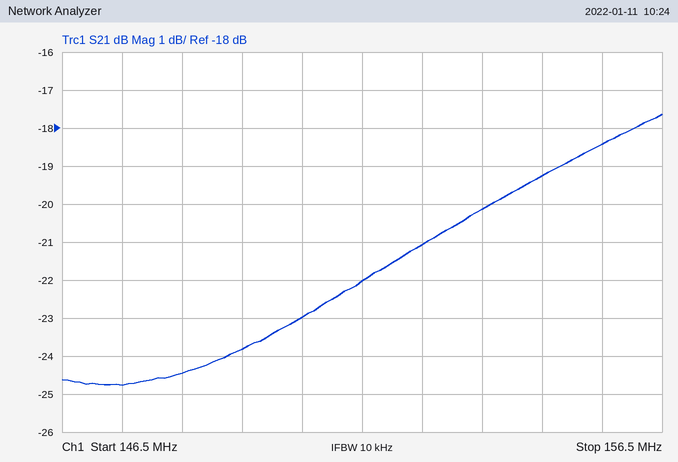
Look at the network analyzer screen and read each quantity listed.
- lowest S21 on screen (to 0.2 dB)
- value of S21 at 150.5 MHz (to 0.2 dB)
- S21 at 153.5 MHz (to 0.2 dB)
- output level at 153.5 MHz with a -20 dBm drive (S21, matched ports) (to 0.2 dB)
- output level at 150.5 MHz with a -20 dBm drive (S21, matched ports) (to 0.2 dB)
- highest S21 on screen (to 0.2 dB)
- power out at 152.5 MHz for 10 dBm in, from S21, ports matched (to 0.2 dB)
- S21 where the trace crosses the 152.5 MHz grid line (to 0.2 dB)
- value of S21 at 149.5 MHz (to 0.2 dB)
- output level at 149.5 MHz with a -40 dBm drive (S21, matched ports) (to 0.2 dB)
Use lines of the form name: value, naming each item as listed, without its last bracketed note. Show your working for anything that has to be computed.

lowest S21 on screen: -24.8 dB
value of S21 at 150.5 MHz: -23.0 dB
S21 at 153.5 MHz: -20.2 dB
output level at 153.5 MHz with a -20 dBm drive (S21, matched ports): -20 dBm + (-20.2 dB) = -40.2 dBm
output level at 150.5 MHz with a -20 dBm drive (S21, matched ports): -20 dBm + (-23.0 dB) = -43.0 dBm
highest S21 on screen: -17.6 dB
power out at 152.5 MHz for 10 dBm in, from S21, ports matched: 10 dBm + (-21.0 dB) = -11.0 dBm
S21 where the trace crosses the 152.5 MHz grid line: -21.0 dB
value of S21 at 149.5 MHz: -23.8 dB
output level at 149.5 MHz with a -40 dBm drive (S21, matched ports): -40 dBm + (-23.8 dB) = -63.8 dBm
